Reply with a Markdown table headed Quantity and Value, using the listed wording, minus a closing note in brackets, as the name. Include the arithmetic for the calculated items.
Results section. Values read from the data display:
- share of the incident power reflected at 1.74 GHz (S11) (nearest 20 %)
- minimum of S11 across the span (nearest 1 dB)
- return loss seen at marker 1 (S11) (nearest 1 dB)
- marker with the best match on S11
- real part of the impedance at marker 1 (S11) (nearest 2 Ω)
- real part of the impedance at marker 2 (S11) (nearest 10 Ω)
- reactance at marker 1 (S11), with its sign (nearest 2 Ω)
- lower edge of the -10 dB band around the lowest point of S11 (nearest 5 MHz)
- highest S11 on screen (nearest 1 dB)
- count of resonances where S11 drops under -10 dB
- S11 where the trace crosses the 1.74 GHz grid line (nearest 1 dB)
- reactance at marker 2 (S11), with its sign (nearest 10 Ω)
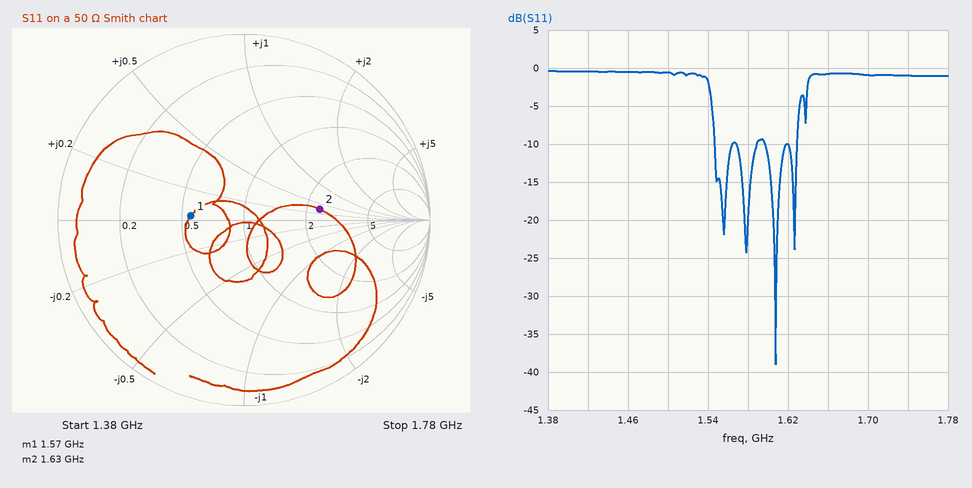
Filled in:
| Quantity | Value |
|---|---|
| share of the incident power reflected at 1.74 GHz (S11) | 10^(-1/10) ≈ 79.4 %, so 80 % to the nearest 20 % |
| minimum of S11 across the span | -39 dB |
| return loss seen at marker 1 (S11) | 11 dB |
| marker with the best match on S11 | marker 1 |
| real part of the impedance at marker 1 (S11) | 28 Ω |
| real part of the impedance at marker 2 (S11) | 120 Ω |
| reactance at marker 1 (S11), with its sign | +2 Ω |
| lower edge of the -10 dB band around the lowest point of S11 | 1.595 GHz |
| highest S11 on screen | 0 dB |
| count of resonances where S11 drops under -10 dB | 4 |
| S11 where the trace crosses the 1.74 GHz grid line | -1 dB |
| reactance at marker 2 (S11), with its sign | +20 Ω |
